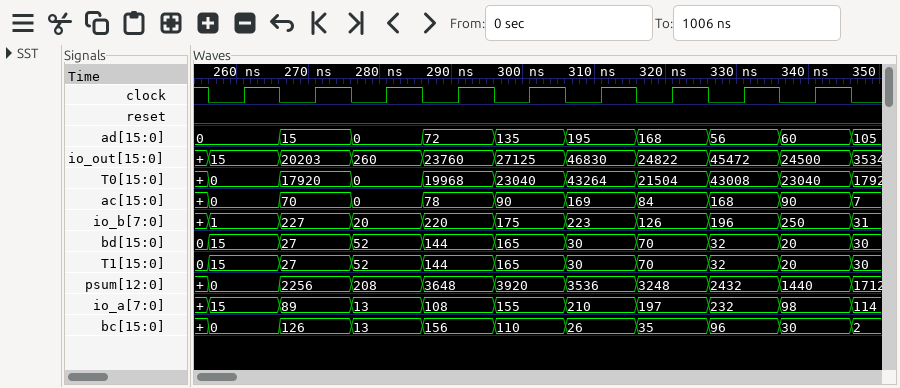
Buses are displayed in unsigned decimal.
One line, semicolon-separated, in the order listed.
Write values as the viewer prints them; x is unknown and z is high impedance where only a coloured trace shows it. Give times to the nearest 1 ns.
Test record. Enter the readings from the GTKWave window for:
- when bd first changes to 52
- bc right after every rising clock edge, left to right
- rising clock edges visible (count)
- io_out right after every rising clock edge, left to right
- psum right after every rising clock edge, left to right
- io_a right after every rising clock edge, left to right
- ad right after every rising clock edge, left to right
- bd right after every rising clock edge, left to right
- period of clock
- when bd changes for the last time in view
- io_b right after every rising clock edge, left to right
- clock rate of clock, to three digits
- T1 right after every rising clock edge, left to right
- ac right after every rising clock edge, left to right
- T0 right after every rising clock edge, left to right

276 ns; 0, 126, 13, 156, 110, 26, 35, 96, 30; 9; 15, 20203, 260, 23760, 27125, 46830, 24822, 45472, 24500; 0, 2256, 208, 3648, 3920, 3536, 3248, 2432, 1440; 15, 89, 13, 108, 155, 210, 197, 232, 98; 0, 15, 0, 72, 135, 195, 168, 56, 60; 15, 27, 52, 144, 165, 30, 70, 32, 20; 10 ns; 346 ns; 1, 227, 20, 220, 175, 223, 126, 196, 250; 100 MHz; 15, 27, 52, 144, 165, 30, 70, 32, 20; 0, 70, 0, 78, 90, 169, 84, 168, 90; 0, 17920, 0, 19968, 23040, 43264, 21504, 43008, 23040
